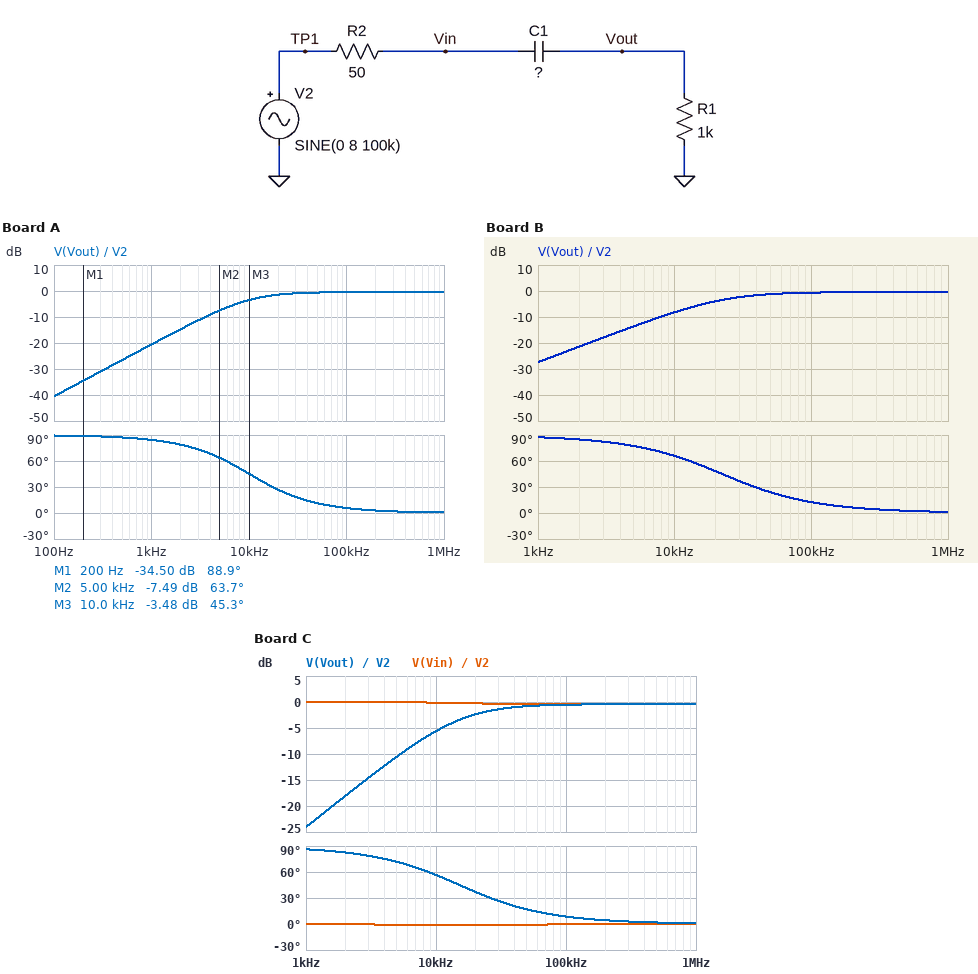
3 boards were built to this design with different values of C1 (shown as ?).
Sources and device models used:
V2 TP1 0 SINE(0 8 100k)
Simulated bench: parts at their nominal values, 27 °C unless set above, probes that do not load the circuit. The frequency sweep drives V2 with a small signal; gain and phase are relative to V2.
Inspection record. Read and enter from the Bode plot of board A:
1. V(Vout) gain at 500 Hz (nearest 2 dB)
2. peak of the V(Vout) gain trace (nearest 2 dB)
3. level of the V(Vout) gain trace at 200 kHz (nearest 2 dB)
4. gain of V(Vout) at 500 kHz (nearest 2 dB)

-26 dB
0 dB
0 dB
0 dB
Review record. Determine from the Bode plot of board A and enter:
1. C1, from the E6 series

15 nF
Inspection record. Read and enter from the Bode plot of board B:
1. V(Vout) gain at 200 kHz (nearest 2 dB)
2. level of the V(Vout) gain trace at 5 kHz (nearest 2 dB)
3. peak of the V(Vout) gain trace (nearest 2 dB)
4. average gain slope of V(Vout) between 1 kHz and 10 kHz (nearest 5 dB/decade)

0 dB
-14 dB
0 dB
20 dB/decade
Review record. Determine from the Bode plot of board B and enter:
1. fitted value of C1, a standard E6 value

6.8 nF
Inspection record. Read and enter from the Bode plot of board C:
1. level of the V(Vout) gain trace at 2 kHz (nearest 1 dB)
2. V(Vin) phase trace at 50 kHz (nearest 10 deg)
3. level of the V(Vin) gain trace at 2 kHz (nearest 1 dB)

-18 dB
0 deg
0 dB
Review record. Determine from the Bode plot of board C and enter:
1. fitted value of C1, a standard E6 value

10 nF
